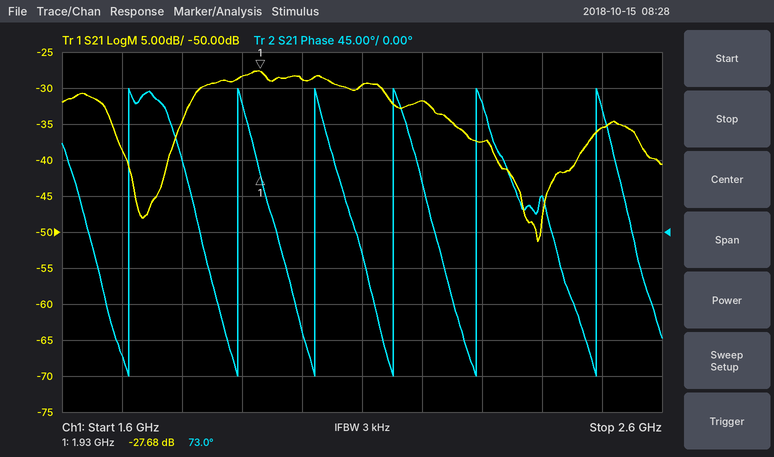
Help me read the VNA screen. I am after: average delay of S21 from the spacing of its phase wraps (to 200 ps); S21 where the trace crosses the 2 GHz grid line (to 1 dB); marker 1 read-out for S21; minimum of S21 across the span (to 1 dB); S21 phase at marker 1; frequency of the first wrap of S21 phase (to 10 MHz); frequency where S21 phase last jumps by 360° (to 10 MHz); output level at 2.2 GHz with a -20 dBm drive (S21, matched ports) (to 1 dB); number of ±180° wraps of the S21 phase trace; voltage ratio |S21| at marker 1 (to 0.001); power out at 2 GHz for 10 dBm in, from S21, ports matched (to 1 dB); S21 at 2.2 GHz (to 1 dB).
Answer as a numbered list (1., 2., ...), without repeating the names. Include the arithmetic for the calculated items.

1. 5 cycles / (2.49 GHz − 1.71 GHz) ≈ 6.4 ns
2. -29 dB
3. -27.68 dB
4. -51 dB
5. 73.0°
6. 1.71 GHz
7. 2.49 GHz
8. -20 dBm + (-32 dB) = -52 dBm
9. 6
10. 10^(-27.68/20) ≈ 0.041
11. 10 dBm + (-29 dB) = -19 dBm
12. -32 dB
